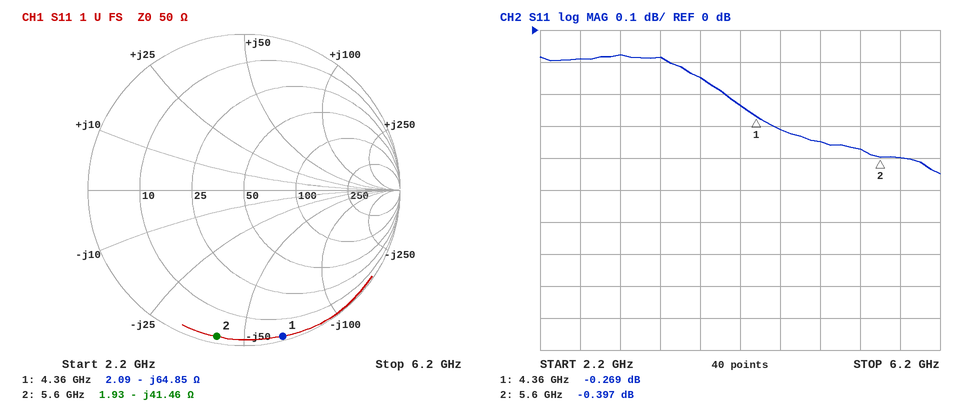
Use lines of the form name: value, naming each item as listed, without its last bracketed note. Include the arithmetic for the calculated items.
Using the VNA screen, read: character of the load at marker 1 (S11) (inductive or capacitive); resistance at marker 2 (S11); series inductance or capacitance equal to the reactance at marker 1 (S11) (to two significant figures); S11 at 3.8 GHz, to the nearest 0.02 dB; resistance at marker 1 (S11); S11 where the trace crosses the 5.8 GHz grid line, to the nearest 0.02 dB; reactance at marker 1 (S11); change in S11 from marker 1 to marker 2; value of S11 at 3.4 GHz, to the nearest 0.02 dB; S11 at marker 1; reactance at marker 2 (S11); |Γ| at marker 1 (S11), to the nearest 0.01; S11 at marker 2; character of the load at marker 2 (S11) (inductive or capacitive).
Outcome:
character of the load at marker 1 (S11): capacitive
resistance at marker 2: 1.93 Ω
series inductance or capacitance equal to the reactance at marker 1 (S11): C = 1/(2π × 4.36 GHz × 64.85 Ω) ≈ 563 fF, so 560 fF to two significant figures
S11 at 3.8 GHz, to the nearest 0.02 dB: -0.14 dB
resistance at marker 1: 2.09 Ω
S11 where the trace crosses the 5.8 GHz grid line, to the nearest 0.02 dB: -0.40 dB
reactance at marker 1: -64.85 Ω
change in S11 from marker 1 to marker 2: -0.397 − (-0.269) = -0.128 dB
value of S11 at 3.4 GHz, to the nearest 0.02 dB: -0.08 dB
S11 at marker 1: -0.269 dB
reactance at marker 2: -41.46 Ω
|Γ| at marker 1 (S11), to the nearest 0.01: 0.97
S11 at marker 2: -0.397 dB
character of the load at marker 2 (S11): capacitive
